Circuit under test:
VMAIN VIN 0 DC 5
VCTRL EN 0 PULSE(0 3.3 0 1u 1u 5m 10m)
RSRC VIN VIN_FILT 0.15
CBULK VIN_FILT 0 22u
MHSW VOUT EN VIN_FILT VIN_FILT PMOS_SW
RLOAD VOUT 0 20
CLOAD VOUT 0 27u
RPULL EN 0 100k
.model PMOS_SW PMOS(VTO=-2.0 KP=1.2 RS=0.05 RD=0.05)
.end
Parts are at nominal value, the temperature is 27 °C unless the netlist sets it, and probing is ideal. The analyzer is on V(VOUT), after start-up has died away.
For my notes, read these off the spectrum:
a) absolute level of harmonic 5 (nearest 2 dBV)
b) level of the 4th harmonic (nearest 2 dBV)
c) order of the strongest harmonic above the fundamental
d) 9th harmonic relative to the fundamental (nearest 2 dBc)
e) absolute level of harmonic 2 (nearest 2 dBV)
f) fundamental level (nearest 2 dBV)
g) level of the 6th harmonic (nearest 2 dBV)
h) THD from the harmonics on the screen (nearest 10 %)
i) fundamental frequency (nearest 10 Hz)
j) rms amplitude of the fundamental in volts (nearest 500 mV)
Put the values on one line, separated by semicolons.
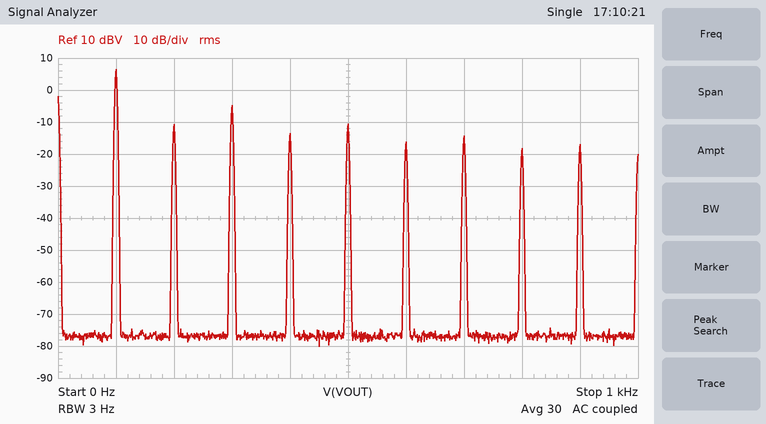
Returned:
-10 dBV; -14 dBV; 3; -24 dBc; -10 dBV; 6 dBV; -16 dBV; 40 %; 100 Hz; 2.0 V
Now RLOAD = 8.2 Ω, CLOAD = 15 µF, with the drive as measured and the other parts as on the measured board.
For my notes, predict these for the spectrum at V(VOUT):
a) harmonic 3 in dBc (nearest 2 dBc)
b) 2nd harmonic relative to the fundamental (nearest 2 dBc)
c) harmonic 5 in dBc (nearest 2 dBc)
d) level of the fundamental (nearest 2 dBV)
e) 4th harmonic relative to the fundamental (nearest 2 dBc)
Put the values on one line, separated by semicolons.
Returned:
-10 dBc; -30 dBc; -14 dBc; 6 dBV; -30 dBc
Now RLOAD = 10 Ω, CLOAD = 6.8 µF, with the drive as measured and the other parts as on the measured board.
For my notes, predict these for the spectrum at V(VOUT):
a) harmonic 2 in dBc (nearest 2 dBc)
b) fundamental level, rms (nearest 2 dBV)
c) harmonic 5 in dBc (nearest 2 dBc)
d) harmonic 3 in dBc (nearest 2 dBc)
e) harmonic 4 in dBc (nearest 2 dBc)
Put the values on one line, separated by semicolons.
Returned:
-34 dBc; 6 dBV; -14 dBc; -10 dBc; -34 dBc
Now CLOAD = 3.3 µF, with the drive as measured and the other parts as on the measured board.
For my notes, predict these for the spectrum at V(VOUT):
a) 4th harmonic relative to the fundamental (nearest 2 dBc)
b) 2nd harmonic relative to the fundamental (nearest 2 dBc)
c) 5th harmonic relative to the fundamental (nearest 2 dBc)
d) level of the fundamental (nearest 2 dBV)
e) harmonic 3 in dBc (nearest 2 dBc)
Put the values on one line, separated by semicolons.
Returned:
-34 dBc; -34 dBc; -14 dBc; 6 dBV; -10 dBc
